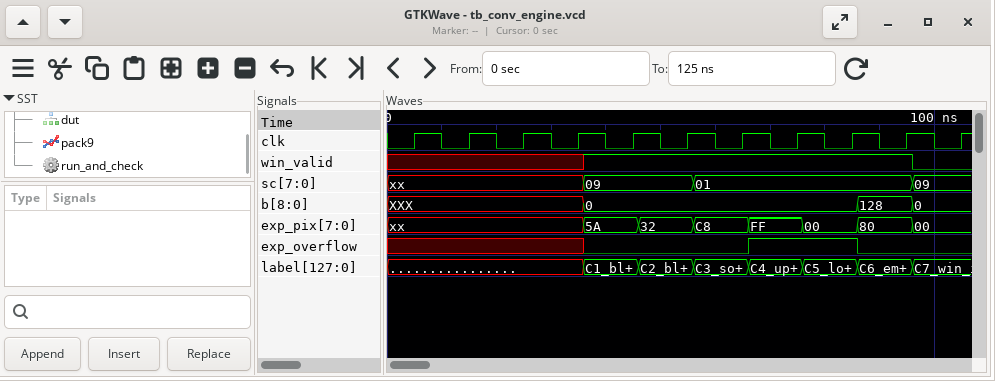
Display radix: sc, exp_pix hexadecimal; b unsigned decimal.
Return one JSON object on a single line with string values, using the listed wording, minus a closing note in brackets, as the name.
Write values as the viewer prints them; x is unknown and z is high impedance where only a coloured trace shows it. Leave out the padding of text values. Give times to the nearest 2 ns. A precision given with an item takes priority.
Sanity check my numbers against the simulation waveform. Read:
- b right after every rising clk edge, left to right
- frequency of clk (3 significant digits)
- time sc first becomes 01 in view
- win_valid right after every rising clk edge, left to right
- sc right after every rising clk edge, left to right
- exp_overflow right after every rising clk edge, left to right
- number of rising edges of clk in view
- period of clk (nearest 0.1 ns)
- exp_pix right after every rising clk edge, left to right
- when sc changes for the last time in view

{"b right after every rising clk edge, left to right": "XXX, XXX, XXX, XXX, 0, 0, 0, 0, 0, 128, 0", "frequency of clk": "100 MHz", "time sc first becomes 01 in view": "56 ns", "win_valid right after every rising clk edge, left to right": "x x x x 1 1 1 1 1 1 0", "sc right after every rising clk edge, left to right": "xx, xx, xx, xx, 09, 09, 01, 01, 01, 01, 09", "exp_overflow right after every rising clk edge, left to right": "x x x x 0 0 0 1 1 0 0", "number of rising edges of clk in view": "11", "period of clk": "10 ns", "exp_pix right after every rising clk edge, left to right": "xx, xx, xx, xx, 5A, 32, C8, FF, 00, 80, 00", "when sc changes for the last time in view": "96 ns"}
